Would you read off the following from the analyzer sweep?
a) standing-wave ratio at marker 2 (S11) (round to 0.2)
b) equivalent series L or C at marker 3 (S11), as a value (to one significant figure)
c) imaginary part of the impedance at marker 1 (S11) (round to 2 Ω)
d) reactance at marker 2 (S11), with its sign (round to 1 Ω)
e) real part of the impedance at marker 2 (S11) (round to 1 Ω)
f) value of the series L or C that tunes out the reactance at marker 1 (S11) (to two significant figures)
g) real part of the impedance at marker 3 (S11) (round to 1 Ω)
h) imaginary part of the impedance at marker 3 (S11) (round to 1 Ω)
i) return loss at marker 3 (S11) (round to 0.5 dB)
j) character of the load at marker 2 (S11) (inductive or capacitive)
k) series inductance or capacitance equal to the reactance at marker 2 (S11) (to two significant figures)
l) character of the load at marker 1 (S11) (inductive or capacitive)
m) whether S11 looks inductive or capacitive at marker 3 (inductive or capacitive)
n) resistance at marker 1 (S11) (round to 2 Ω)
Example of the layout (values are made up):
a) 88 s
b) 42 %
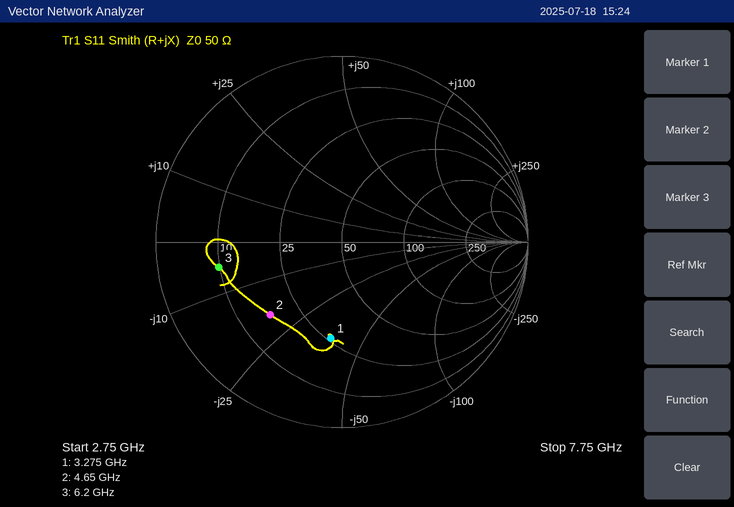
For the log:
a) 3.4
b) 5 pF
c) -38 Ω
d) -19 Ω
e) 17 Ω
f) 1.8 nH
g) 10 Ω
h) -5 Ω
i) 3.5 dB
j) capacitive
k) 1.8 pF
l) capacitive
m) capacitive
n) 26 Ω
